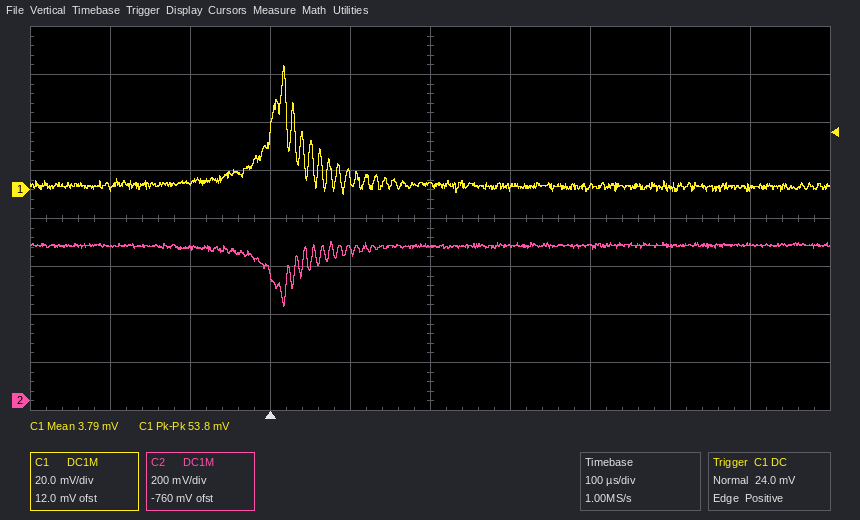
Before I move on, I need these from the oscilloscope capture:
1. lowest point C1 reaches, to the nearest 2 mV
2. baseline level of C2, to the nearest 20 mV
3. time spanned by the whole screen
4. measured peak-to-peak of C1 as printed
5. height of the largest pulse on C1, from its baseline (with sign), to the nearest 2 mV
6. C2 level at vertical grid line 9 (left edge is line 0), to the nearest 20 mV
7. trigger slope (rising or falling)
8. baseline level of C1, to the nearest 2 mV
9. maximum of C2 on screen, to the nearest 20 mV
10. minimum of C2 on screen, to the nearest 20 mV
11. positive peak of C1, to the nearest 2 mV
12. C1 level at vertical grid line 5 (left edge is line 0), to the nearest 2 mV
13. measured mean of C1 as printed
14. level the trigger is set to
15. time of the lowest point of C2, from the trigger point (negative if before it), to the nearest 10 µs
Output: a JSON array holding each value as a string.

["-2 mV", "640 mV", "1 ms", "53.8 mV", "+50 mV", "660 mV", "rising", "2 mV", "660 mV", "400 mV", "52 mV", "2 mV", "3.79 mV", "24.0 mV", "+20 µs"]
